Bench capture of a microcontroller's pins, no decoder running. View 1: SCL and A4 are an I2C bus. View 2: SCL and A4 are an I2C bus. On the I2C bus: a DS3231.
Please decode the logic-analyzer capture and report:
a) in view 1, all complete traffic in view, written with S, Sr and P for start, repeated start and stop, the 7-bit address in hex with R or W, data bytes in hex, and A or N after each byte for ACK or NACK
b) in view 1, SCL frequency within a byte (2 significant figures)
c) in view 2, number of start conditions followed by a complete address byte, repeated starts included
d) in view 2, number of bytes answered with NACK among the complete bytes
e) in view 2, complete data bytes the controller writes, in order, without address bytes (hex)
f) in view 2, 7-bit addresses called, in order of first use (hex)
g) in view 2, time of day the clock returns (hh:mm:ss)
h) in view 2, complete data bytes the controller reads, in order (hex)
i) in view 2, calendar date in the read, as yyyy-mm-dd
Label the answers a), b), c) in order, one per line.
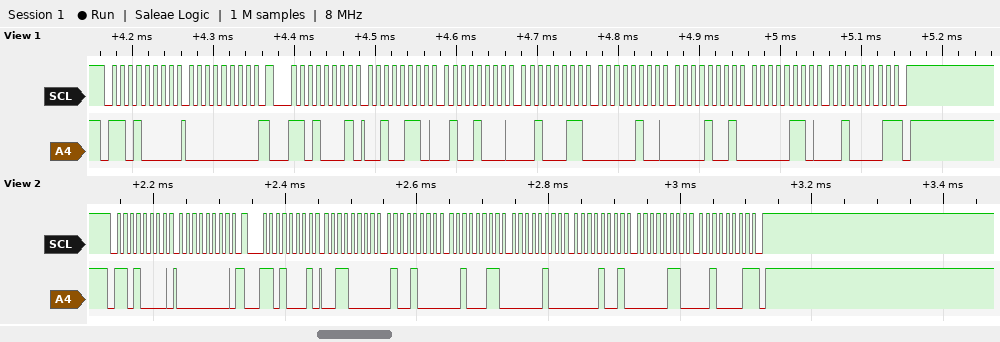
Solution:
a) S 68W A 00 A Sr 68R A 26 A 48 A 23 A 04 A 09 A 06 A 21 N P
b) 100 kHz
c) 2
d) 1
e) 00
f) 0x68
g) 23:48:30
h) 30 48 23 04 09 06 21
i) 2021-06-09
